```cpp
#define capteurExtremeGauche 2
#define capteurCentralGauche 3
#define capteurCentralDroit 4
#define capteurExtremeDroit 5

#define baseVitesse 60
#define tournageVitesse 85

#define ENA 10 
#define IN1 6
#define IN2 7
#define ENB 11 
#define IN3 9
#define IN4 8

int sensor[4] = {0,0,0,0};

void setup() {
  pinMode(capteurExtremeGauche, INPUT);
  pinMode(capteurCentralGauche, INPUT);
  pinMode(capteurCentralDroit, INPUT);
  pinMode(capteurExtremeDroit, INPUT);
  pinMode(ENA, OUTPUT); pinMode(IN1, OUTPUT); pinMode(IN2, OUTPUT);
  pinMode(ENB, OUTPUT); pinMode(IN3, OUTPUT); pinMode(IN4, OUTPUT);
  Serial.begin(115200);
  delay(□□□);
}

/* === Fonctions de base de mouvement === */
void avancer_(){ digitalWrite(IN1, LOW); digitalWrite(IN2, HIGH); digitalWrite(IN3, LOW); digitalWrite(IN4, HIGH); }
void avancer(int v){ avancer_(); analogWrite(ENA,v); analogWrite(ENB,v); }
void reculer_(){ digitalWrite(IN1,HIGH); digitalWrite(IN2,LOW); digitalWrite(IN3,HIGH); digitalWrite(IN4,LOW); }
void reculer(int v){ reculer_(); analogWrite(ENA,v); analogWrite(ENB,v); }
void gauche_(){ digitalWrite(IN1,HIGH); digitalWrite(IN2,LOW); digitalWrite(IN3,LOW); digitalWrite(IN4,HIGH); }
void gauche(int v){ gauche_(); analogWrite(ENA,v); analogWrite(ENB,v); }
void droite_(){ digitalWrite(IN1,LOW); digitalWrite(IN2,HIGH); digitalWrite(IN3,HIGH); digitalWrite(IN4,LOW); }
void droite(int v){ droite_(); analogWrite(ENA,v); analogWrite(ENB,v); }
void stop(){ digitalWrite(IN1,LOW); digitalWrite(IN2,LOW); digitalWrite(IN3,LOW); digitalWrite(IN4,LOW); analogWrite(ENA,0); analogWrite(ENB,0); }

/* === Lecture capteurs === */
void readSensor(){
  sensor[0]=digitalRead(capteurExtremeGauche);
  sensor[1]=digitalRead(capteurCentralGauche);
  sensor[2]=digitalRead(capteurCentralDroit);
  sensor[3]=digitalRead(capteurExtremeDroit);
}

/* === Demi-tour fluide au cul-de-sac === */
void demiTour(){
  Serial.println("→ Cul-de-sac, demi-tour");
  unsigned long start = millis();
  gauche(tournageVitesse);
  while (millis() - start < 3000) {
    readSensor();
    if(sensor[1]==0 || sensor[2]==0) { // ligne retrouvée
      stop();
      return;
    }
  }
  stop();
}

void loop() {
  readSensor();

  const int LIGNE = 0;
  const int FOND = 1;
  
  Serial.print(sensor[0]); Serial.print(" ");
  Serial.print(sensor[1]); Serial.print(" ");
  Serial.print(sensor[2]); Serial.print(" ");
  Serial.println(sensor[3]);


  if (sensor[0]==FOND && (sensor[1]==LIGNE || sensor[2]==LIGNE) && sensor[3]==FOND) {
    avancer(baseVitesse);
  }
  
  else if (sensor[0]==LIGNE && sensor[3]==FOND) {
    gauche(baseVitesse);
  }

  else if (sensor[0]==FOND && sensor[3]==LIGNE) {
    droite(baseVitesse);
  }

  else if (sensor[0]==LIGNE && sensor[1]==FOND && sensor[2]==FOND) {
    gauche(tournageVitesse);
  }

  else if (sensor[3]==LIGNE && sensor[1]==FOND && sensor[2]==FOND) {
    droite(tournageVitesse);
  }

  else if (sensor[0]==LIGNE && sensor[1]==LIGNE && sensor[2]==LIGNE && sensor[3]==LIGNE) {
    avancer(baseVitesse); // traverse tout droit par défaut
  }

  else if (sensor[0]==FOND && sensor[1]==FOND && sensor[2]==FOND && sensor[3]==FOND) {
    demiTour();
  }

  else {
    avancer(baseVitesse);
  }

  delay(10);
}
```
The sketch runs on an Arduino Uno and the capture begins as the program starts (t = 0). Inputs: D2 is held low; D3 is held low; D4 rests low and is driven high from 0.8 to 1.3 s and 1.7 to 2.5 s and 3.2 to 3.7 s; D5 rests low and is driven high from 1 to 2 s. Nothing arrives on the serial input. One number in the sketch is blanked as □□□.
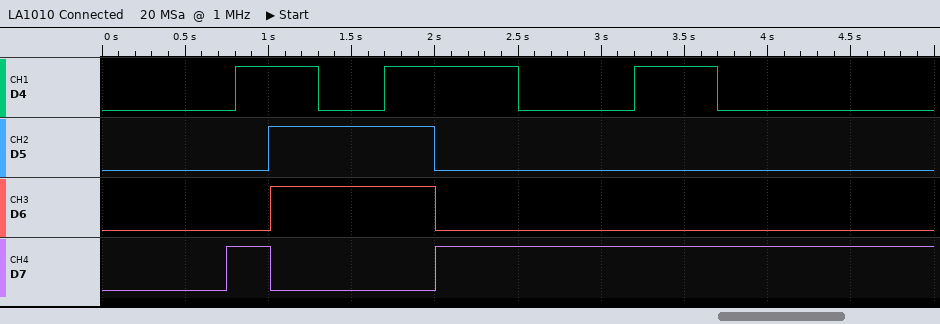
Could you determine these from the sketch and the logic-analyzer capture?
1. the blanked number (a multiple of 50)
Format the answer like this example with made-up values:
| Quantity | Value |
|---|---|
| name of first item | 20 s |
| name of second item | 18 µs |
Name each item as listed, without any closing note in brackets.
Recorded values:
| Quantity | Value |
|---|---|
| the blanked number | 750 |
